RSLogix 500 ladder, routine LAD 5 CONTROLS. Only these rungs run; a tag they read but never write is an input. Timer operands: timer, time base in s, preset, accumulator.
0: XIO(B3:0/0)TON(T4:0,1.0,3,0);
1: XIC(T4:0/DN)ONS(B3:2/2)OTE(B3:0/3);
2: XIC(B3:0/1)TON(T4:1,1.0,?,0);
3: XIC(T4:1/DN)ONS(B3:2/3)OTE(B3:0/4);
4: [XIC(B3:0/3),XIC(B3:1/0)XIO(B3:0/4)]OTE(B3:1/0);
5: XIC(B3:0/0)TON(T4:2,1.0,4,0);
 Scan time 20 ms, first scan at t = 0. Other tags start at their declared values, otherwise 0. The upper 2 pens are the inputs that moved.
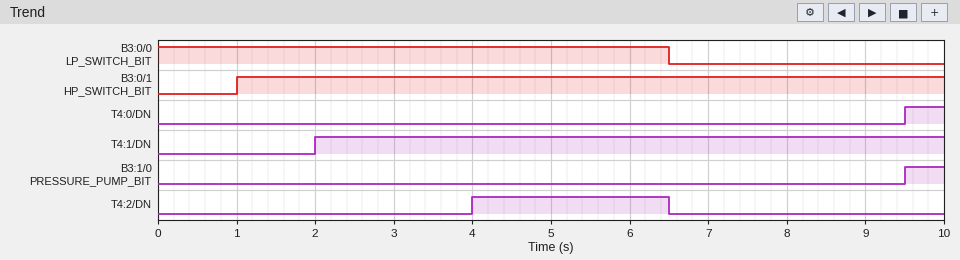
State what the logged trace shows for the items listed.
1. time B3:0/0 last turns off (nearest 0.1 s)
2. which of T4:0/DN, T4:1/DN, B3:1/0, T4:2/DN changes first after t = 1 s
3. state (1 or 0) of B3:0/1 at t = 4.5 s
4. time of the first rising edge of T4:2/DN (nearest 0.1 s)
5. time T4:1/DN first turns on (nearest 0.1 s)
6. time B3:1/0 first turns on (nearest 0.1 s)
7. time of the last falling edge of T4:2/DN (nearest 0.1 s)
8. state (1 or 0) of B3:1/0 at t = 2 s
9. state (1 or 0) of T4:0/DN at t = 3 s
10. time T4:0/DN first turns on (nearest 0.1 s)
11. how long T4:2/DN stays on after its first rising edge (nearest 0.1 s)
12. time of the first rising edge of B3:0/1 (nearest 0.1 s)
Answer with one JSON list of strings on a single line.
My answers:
["6.5 s", "T4:1/DN", "1", "4.0 s", "2.0 s", "9.5 s", "6.5 s", "0", "0", "9.5 s", "2.5 s", "1.0 s"]
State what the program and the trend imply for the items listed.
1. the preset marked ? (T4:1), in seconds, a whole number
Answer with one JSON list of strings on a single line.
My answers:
["1 s"]
